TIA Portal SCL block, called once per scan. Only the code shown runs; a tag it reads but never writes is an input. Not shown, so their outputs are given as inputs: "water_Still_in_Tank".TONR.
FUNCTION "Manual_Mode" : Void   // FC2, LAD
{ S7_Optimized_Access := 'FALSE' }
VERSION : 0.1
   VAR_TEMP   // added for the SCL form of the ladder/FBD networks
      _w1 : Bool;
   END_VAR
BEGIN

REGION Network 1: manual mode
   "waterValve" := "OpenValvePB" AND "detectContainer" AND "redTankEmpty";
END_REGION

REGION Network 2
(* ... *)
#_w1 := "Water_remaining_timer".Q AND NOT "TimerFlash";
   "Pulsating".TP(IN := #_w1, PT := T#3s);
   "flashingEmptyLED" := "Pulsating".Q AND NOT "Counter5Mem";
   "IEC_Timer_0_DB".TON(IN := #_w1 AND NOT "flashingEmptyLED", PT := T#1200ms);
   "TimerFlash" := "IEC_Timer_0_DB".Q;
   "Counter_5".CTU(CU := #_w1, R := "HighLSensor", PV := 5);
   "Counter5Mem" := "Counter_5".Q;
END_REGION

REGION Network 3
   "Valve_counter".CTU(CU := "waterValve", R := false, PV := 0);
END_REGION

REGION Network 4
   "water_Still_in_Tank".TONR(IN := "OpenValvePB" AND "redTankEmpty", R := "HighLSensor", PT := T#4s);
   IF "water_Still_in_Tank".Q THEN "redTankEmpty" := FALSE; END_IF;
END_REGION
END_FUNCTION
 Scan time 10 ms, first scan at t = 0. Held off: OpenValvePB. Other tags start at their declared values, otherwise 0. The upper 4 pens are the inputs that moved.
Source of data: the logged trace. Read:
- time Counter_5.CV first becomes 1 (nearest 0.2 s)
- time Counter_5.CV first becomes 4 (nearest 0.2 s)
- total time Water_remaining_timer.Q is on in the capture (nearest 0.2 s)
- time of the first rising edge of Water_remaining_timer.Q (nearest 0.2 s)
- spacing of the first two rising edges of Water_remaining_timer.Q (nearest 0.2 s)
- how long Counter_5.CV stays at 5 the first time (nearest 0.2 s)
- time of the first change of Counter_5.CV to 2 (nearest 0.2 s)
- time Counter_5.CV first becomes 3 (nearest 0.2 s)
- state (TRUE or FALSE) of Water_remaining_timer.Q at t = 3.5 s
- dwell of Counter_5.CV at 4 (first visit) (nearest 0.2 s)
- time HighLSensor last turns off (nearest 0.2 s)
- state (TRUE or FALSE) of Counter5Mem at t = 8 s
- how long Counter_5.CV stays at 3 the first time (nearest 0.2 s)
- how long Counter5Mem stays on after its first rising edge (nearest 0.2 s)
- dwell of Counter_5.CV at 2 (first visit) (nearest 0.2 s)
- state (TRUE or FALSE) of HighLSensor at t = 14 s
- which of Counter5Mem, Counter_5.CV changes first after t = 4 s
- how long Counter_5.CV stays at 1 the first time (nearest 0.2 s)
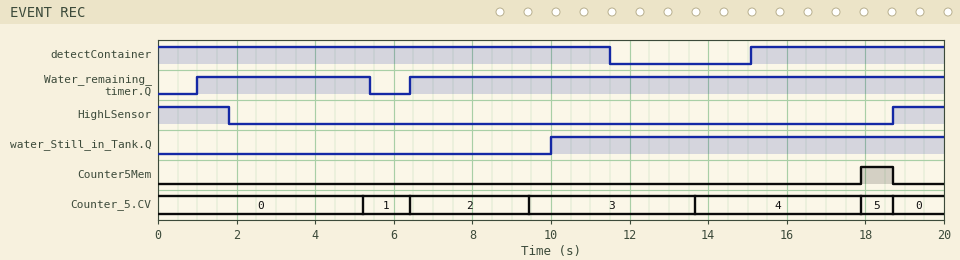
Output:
5.2 s
13.6 s
18.0 s
1.0 s
5.4 s
0.8 s
6.4 s
9.4 s
TRUE
4.2 s
1.8 s
FALSE
4.2 s
0.8 s
3.0 s
FALSE
Counter_5.CV
1.2 s
